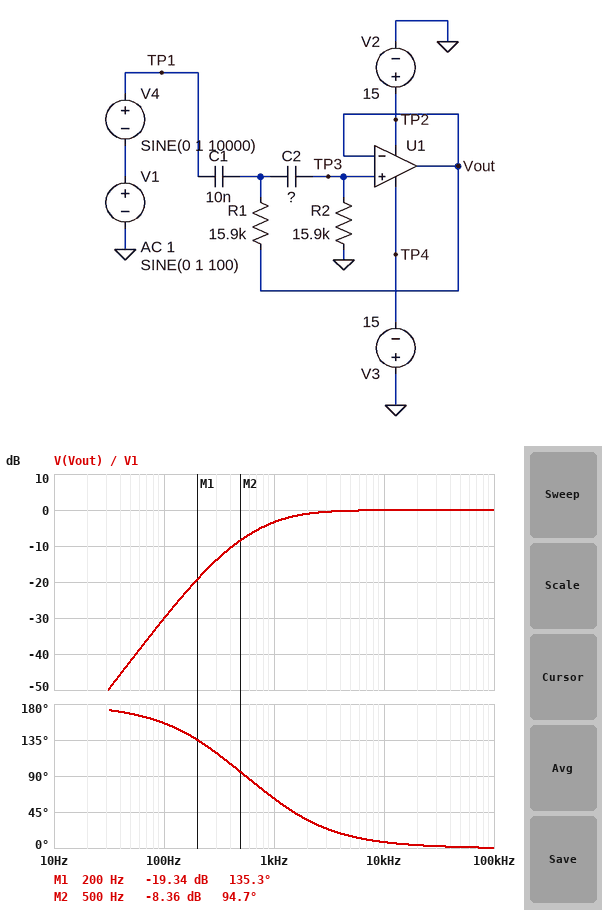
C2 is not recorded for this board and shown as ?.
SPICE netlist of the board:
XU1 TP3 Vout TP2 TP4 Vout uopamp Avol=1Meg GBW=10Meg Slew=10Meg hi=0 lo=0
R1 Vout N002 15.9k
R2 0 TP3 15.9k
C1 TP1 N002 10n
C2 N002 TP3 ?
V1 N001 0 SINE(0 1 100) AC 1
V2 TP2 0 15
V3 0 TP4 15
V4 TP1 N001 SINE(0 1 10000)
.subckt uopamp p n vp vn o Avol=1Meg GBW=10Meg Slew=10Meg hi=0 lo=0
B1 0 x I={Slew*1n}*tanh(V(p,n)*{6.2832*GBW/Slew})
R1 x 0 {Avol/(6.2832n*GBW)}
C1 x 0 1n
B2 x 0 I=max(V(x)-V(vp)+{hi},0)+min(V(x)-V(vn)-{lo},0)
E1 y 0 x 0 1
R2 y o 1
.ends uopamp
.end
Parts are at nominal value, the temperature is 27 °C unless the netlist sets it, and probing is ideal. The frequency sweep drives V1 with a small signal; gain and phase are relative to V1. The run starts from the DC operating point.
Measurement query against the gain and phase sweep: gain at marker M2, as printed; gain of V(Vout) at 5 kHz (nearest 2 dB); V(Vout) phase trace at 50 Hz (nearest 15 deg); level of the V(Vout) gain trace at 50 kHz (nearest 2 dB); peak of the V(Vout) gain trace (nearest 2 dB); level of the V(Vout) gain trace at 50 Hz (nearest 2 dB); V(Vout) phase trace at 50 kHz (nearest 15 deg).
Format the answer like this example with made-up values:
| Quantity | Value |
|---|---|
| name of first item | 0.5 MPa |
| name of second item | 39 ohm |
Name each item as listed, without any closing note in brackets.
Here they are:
| Quantity | Value |
|---|---|
| gain at marker M2, as printed | -8.36 dB |
| gain of V(Vout) at 5 kHz | 0 dB |
| V(Vout) phase trace at 50 Hz | 165 deg |
| level of the V(Vout) gain trace at 50 kHz | 0 dB |
| peak of the V(Vout) gain trace | 0 dB |
| level of the V(Vout) gain trace at 50 Hz | -42 dB |
| V(Vout) phase trace at 50 kHz | 0 deg |
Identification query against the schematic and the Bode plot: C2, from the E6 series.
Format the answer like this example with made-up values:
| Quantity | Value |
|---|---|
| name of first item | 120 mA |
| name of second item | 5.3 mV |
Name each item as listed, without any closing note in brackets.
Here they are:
| Quantity | Value |
|---|---|
| C2, from the E6 series | 33 nF |
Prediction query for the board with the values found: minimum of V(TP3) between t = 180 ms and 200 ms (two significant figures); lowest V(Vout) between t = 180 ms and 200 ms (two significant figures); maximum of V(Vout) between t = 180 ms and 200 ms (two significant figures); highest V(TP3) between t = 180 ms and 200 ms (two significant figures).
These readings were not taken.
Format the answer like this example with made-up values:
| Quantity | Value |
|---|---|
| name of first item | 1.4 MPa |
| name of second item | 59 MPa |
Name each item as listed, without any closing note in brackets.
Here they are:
| Quantity | Value |
|---|---|
| minimum of V(TP3) between t = 180 ms and 200 ms | -1.0 V |
| lowest V(Vout) between t = 180 ms and 200 ms | -1.0 V |
| maximum of V(Vout) between t = 180 ms and 200 ms | 1.0 V |
| highest V(TP3) between t = 180 ms and 200 ms | 1.0 V |
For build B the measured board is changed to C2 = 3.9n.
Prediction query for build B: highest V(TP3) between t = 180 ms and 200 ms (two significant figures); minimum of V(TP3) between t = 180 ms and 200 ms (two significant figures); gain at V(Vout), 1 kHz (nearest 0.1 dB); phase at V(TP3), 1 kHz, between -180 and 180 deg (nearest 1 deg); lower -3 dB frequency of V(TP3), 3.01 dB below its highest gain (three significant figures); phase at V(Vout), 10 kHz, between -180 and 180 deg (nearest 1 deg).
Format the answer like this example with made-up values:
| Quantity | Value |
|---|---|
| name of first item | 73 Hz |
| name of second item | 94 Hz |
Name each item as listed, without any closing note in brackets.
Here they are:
| Quantity | Value |
|---|---|
| highest V(TP3) between t = 180 ms and 200 ms | 970 mV |
| minimum of V(TP3) between t = 180 ms and 200 ms | -970 mV |
| gain at V(Vout), 1 kHz | -11.8 dB |
| phase at V(TP3), 1 kHz, between -180 and 180 deg | 114 deg |
| lower -3 dB frequency of V(TP3), 3.01 dB below its highest gain | 2.89 kHz |
| phase at V(Vout), 10 kHz, between -180 and 180 deg | 20 deg |
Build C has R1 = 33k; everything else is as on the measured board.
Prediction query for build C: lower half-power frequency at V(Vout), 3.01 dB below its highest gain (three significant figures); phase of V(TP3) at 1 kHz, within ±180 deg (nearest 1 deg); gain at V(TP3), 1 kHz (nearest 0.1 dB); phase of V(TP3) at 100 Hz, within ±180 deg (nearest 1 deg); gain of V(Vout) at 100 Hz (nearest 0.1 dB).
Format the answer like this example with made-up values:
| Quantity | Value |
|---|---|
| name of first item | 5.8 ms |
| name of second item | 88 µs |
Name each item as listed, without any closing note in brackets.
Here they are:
| Quantity | Value |
|---|---|
| lower half-power frequency at V(Vout), 3.01 dB below its highest gain | 1.19 kHz |
| phase of V(TP3) at 1 kHz, within ±180 deg | 57 deg |
| gain at V(TP3), 1 kHz | -3.9 dB |
| phase of V(TP3) at 100 Hz, within ±180 deg | 136 deg |
| gain of V(Vout) at 100 Hz | -25.5 dB |
